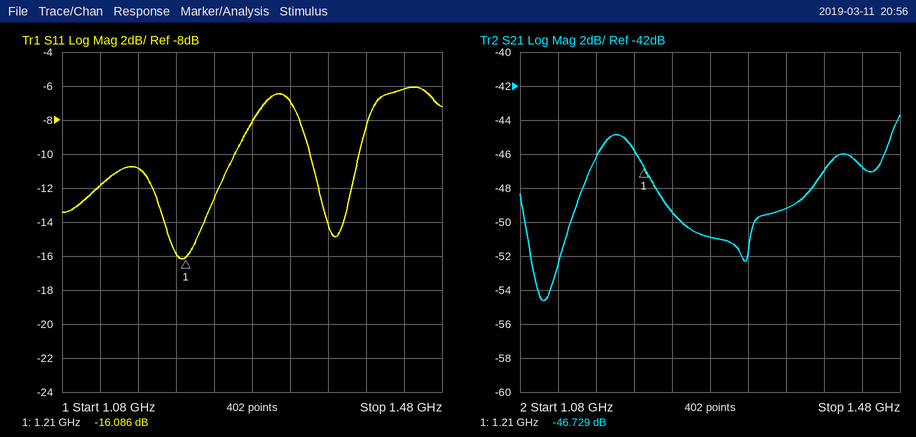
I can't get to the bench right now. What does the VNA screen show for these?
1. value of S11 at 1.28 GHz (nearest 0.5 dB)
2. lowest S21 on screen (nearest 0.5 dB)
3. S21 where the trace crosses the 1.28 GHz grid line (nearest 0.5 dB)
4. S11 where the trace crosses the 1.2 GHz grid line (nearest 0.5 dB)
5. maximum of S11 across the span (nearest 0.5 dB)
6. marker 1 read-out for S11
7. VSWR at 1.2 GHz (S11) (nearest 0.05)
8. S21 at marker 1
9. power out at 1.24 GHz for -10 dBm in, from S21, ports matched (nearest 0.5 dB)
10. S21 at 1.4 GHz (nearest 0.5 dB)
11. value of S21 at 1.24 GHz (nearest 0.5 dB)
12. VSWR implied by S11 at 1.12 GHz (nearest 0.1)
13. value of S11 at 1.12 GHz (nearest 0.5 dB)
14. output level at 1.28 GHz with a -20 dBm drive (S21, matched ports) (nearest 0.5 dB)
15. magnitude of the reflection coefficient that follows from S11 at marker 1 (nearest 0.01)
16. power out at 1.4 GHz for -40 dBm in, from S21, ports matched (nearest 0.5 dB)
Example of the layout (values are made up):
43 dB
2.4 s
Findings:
-8.0 dB
-54.5 dB
-51.0 dB
-16.0 dB
-6.0 dB
-16.086 dB
1.40
-46.729 dB
-59.5 dBm
-47.0 dB
-49.5 dB
1.7
-12.0 dB
-71.0 dBm
0.16
-87.0 dBm
